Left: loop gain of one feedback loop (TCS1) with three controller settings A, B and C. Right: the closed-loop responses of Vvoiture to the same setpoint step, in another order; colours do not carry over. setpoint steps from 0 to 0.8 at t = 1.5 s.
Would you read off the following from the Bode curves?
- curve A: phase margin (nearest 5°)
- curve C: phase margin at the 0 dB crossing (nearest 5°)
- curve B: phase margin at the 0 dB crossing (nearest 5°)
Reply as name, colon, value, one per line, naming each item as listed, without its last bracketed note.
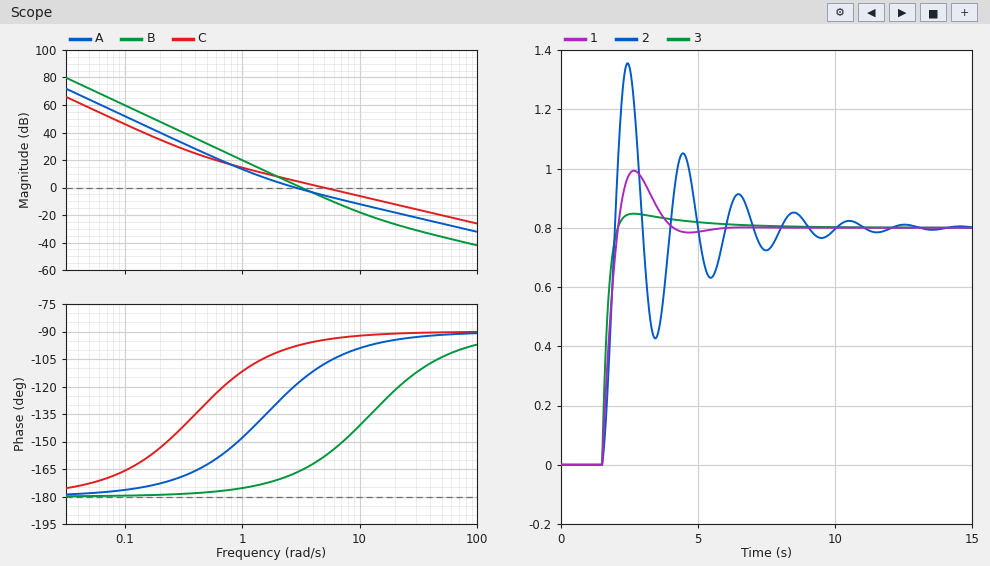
curve A: phase margin: 60°
curve C: phase margin at the 0 dB crossing: 85°
curve B: phase margin at the 0 dB crossing: 15°
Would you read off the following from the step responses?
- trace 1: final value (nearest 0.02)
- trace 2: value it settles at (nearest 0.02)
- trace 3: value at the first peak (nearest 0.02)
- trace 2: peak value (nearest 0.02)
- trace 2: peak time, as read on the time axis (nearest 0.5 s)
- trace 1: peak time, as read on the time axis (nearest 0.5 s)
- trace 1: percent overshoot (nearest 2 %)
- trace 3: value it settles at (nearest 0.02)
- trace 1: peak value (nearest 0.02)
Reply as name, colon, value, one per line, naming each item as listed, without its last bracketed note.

trace 1: final value: 0.80
trace 2: value it settles at: 0.80
trace 3: value at the first peak: 0.84
trace 2: peak value: 1.36
trace 2: peak time, as read on the time axis: 2.5 s
trace 1: peak time, as read on the time axis: 2.5 s
trace 1: percent overshoot: 24 %
trace 3: value it settles at: 0.80
trace 1: peak value: 1.00
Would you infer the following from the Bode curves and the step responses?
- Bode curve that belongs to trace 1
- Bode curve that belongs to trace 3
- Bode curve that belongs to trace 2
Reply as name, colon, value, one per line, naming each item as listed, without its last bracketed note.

Bode curve that belongs to trace 1: A
Bode curve that belongs to trace 3: C
Bode curve that belongs to trace 2: B
